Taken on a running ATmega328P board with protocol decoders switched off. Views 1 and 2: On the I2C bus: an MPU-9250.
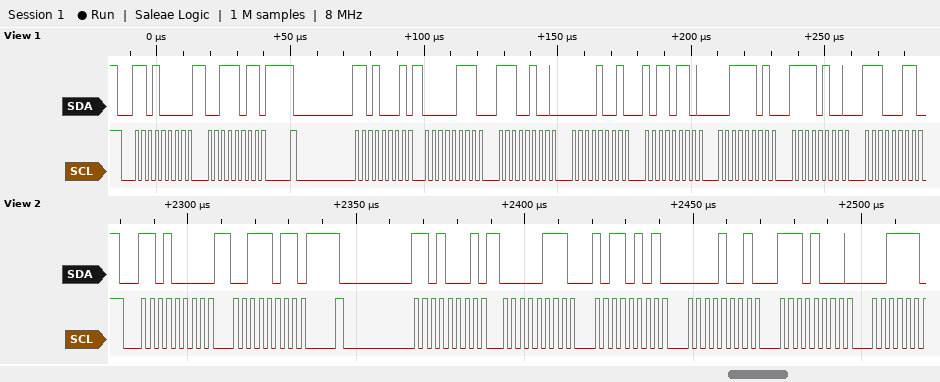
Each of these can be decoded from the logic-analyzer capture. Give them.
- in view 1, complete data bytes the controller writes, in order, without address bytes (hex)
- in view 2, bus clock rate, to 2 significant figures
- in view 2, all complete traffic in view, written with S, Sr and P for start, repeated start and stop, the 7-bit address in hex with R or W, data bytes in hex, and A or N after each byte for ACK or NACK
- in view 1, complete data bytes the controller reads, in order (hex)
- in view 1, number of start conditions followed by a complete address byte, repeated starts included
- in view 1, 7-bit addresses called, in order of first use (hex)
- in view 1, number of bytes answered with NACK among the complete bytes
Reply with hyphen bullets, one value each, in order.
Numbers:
- 3B
- 400 kHz
- S 68W A 3B A Sr 68R A 07 A B5 A 09 A E8 A
- 07 E4 09 B6 3D F4 E3
- 2
- 0x68
- 0
